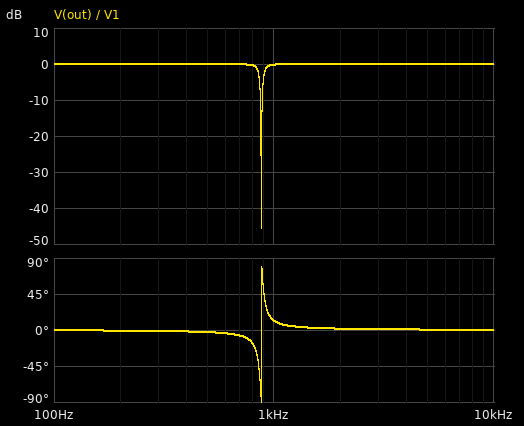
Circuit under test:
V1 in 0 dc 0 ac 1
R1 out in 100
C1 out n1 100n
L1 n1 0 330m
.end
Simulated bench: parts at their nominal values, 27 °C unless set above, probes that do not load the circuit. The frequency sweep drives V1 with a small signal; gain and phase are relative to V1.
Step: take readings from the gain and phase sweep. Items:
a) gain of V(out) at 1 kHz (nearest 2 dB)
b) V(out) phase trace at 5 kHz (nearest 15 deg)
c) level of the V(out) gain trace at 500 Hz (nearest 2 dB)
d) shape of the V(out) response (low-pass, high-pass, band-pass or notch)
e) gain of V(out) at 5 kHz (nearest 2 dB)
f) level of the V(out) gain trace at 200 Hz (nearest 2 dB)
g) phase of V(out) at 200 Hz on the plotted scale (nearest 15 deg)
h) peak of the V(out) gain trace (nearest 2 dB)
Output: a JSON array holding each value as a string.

["0 dB", "0 deg", "0 dB", "notch", "0 dB", "0 dB", "0 deg", "0 dB"]
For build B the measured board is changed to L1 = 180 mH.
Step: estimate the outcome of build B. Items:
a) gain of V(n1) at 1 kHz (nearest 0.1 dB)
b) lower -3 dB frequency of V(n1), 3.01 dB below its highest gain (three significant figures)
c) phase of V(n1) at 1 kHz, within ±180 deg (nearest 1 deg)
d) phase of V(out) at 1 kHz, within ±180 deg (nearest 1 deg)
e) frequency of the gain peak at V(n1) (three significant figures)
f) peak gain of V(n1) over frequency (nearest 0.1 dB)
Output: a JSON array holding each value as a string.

["7.6 dB", "1.15 kHz", "168 deg", "-12 deg", "1.19 kHz", "22.6 dB"]
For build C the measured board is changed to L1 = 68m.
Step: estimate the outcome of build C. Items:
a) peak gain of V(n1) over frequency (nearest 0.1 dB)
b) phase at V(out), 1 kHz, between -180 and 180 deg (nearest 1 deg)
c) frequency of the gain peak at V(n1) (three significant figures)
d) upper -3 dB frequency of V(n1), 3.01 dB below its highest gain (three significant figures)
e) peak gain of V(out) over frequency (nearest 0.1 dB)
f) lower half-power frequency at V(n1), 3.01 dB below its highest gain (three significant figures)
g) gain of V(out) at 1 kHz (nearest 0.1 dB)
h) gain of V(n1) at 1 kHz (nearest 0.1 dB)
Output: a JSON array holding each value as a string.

["18.3 dB", "-5 deg", "1.94 kHz", "2.07 kHz", "0 dB", "1.83 kHz", "0 dB", "-8.7 dB"]
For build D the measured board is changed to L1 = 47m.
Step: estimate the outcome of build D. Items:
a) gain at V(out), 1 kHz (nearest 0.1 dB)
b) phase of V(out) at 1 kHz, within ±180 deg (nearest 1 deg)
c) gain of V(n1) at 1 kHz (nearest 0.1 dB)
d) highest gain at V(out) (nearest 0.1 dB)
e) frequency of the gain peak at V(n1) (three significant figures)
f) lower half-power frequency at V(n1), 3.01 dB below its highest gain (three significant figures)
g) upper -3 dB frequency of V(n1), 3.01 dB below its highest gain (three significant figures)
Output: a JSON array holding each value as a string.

["0 dB", "-4 deg", "-12.9 dB", "0 dB", "2.33 kHz", "2.18 kHz", "2.53 kHz"]
